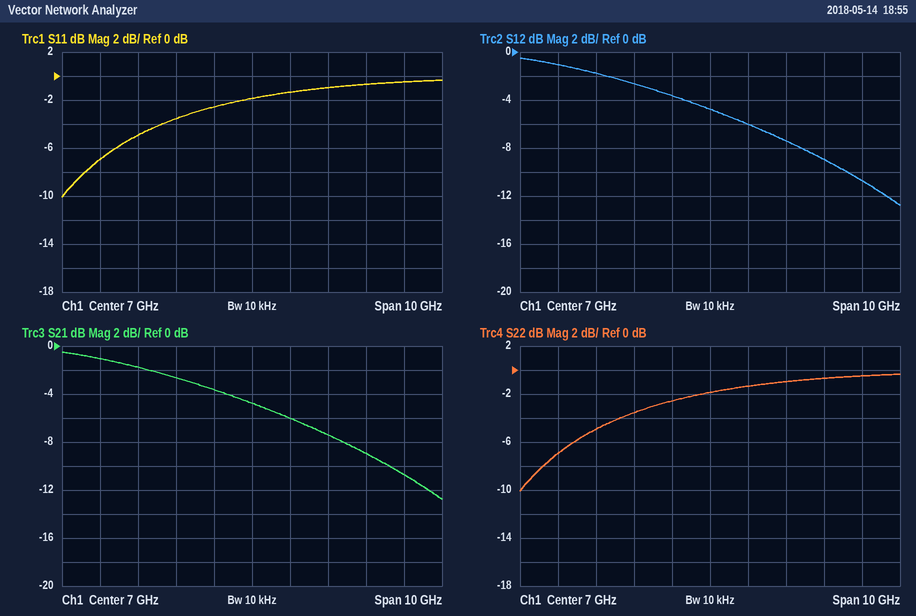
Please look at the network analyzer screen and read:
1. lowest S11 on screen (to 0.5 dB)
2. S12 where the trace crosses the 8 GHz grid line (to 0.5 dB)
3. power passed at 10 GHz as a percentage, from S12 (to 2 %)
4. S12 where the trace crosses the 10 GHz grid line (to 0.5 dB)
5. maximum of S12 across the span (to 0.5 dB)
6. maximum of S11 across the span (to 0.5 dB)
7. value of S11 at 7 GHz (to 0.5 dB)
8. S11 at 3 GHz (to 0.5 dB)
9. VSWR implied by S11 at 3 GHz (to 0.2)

-10.0 dB
-6.0 dB
12 %
-9.0 dB
-0.5 dB
-0.5 dB
-2.0 dB
-7.0 dB
2.6
